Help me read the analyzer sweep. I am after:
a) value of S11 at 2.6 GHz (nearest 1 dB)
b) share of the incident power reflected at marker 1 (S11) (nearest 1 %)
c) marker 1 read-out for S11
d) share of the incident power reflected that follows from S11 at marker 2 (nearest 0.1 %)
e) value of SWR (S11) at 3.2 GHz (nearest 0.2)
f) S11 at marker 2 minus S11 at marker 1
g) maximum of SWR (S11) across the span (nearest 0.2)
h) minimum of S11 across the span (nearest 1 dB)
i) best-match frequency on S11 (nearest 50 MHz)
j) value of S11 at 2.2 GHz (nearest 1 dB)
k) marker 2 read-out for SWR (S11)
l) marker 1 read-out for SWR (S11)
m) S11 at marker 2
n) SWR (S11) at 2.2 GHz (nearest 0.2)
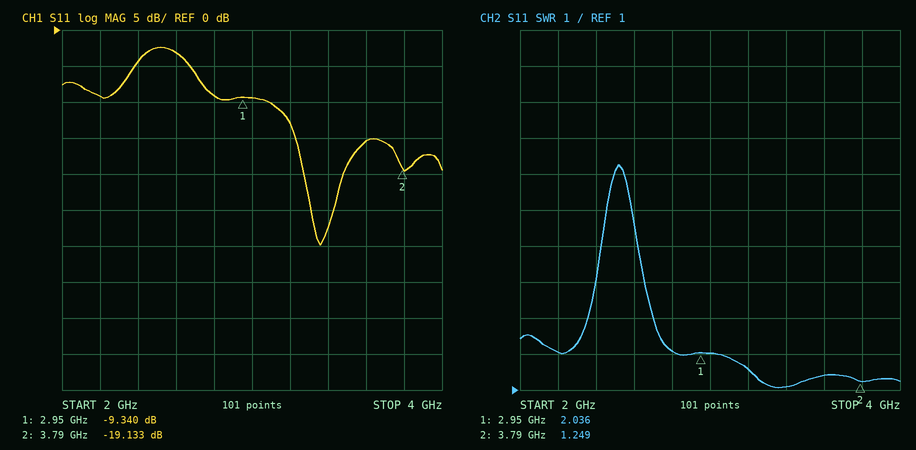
-3 dB
12 %
-9.340 dB
1.2 %
1.6
-9.793 dB
7.2
-30 dB
3.35 GHz
-9 dB
1.249
2.036
-19.133 dB
2.0
